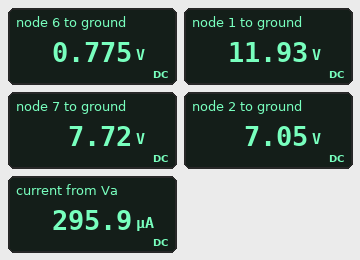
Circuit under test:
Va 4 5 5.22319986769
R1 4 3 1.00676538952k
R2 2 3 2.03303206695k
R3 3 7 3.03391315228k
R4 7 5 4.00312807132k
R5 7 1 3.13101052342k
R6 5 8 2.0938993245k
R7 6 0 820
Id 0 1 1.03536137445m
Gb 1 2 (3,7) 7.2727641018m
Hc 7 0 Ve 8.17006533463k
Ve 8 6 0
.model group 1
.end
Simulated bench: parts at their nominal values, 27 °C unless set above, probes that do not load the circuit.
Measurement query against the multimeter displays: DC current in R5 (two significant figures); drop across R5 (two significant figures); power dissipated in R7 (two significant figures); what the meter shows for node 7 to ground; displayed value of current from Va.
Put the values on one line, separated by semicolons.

1.3 mA; 4.2 V; 730 µW; 7.72 V; 295.9 µA
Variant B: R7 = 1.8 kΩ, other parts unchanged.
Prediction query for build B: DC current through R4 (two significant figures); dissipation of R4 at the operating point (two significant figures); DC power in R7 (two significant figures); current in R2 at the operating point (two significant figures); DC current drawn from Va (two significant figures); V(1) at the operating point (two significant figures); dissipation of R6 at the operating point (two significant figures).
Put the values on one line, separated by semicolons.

1.3 mA; 6.6 mW; 2.6 mW; 86 µA; 82 µA; 13 V; 3.0 mW
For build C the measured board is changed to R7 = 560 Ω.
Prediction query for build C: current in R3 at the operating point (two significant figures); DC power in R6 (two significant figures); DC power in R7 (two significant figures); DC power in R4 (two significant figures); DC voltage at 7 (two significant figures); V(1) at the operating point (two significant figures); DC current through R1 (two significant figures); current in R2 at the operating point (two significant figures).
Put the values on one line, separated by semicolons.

16 µA; 1.7 mW; 450 µW; 6.1 mW; 7.3 V; 12 V; 340 µA; 350 µA
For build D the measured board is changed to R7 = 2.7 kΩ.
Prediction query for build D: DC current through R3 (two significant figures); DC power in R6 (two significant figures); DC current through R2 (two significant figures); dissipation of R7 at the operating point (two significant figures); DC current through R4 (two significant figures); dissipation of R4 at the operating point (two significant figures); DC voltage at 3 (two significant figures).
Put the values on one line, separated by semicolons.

12 µA; 5.4 mW; 260 µA; 7.0 mW; 1.4 mA; 7.4 mW; 13 V
